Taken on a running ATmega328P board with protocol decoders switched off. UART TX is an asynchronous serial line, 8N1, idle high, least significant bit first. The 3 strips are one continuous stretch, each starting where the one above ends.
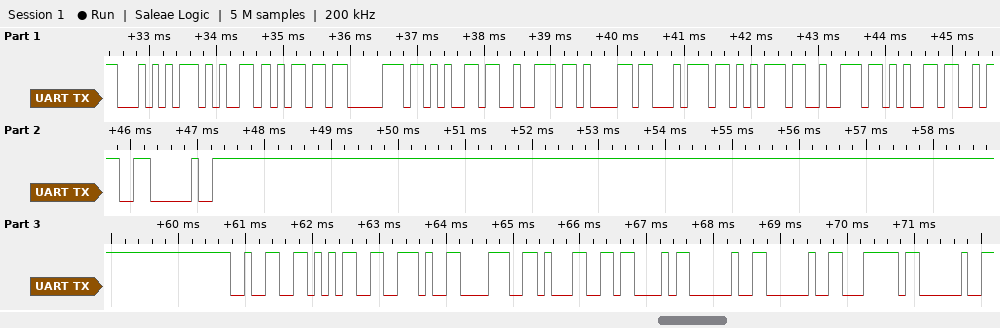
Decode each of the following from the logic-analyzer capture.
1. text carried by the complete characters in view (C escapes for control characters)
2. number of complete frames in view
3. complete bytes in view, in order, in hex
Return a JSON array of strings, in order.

["\"Temperature: 25.81C  | \"", "23", "54 65 6D 70 65 72 61 74 75 72 65 3A 20 32 35 2E 38 31 43 20 20 7C 20"]
